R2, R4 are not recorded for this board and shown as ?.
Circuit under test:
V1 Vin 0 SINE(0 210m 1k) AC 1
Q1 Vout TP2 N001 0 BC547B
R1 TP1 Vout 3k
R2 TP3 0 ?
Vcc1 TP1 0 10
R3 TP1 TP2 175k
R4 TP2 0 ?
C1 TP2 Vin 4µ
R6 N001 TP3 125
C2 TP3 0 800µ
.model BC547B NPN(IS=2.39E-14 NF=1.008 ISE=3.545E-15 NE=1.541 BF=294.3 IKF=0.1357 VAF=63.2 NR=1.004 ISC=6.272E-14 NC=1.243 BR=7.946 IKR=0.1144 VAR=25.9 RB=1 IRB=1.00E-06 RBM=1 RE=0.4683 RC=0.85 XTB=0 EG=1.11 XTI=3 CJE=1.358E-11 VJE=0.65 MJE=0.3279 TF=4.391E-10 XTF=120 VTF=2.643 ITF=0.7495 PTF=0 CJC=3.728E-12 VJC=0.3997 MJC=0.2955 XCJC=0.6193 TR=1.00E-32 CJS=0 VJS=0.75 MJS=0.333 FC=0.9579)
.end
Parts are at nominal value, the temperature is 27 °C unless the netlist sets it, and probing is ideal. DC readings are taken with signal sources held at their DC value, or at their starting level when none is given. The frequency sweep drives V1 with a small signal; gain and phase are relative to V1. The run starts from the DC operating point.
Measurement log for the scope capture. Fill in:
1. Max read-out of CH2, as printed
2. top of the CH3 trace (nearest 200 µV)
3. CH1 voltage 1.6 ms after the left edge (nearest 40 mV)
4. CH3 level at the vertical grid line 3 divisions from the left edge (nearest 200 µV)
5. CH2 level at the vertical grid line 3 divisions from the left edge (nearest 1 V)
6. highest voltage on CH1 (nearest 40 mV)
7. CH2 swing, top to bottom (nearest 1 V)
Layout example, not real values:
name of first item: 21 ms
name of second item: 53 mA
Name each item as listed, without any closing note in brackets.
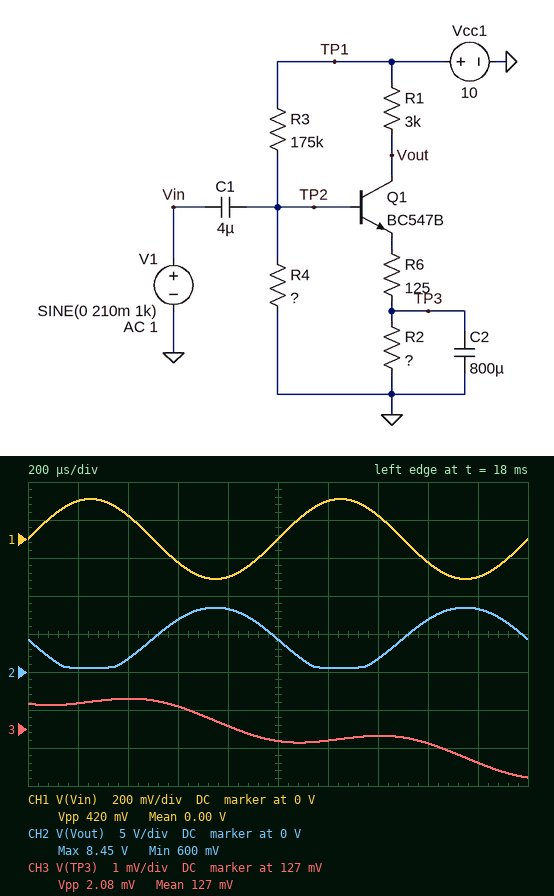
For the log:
Max read-out of CH2, as printed: 8.45 V
top of the CH3 trace: 127.8 mV
CH1 voltage 1.6 ms after the left edge: -120 mV
CH3 level at the vertical grid line 3 divisions from the left edge: 127.6 mV
CH2 level at the vertical grid line 3 divisions from the left edge: 7 V
highest voltage on CH1: 200 mV
CH2 swing, top to bottom: 8 V
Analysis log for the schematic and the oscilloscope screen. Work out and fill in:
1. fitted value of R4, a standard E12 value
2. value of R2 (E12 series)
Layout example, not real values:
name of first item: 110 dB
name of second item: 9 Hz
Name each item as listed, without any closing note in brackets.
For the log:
fitted value of R4, a standard E12 value: 47 kΩ
value of R2: 47 Ω
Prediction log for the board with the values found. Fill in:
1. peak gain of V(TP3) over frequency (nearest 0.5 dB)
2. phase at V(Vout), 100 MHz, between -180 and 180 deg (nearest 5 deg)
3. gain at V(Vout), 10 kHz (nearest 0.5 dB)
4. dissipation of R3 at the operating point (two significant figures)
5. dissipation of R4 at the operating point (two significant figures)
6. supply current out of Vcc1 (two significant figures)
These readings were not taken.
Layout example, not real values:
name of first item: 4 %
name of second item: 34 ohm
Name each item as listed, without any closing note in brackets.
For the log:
peak gain of V(TP3) over frequency: -42.5 dB
phase at V(Vout), 100 MHz, between -180 and 180 deg: 10 deg
gain at V(Vout), 10 kHz: 16.5 dB
dissipation of R3 at the operating point: 440 µW
dissipation of R4 at the operating point: 31 µW
supply current out of Vcc1: 3.2 mA
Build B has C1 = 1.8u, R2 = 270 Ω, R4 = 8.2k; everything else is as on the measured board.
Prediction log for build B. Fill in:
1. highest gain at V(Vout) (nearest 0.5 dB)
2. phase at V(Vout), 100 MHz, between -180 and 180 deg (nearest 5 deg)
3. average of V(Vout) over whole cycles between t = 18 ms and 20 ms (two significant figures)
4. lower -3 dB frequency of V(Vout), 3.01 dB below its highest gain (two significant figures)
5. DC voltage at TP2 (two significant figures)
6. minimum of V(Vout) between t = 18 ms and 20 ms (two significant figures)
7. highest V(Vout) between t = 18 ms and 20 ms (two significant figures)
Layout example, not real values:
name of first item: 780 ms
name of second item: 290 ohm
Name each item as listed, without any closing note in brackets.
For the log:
highest gain at V(Vout): 0 dB
phase at V(Vout), 100 MHz, between -180 and 180 deg: 20 deg
average of V(Vout) over whole cycles between t = 18 ms and 20 ms: 9.8 V
lower -3 dB frequency of V(Vout), 3.01 dB below its highest gain: 34 MHz
DC voltage at TP2: 450 mV
minimum of V(Vout) between t = 18 ms and 20 ms: 8.9 V
highest V(Vout) between t = 18 ms and 20 ms: 10 V
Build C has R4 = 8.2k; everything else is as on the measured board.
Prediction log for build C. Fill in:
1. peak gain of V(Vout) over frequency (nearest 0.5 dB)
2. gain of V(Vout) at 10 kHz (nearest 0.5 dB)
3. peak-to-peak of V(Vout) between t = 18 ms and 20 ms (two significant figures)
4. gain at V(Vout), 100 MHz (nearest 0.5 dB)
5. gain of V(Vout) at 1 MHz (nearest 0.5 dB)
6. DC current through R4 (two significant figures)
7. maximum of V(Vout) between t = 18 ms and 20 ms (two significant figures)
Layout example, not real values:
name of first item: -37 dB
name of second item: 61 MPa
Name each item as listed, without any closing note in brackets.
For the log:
peak gain of V(Vout) over frequency: 0 dB
gain of V(Vout) at 10 kHz: -21.0 dB
peak-to-peak of V(Vout) between t = 18 ms and 20 ms: 1.1 V
gain at V(Vout), 100 MHz: -0.5 dB
gain of V(Vout) at 1 MHz: -20.5 dB
DC current through R4: 55 µA
maximum of V(Vout) between t = 18 ms and 20 ms: 10 V
